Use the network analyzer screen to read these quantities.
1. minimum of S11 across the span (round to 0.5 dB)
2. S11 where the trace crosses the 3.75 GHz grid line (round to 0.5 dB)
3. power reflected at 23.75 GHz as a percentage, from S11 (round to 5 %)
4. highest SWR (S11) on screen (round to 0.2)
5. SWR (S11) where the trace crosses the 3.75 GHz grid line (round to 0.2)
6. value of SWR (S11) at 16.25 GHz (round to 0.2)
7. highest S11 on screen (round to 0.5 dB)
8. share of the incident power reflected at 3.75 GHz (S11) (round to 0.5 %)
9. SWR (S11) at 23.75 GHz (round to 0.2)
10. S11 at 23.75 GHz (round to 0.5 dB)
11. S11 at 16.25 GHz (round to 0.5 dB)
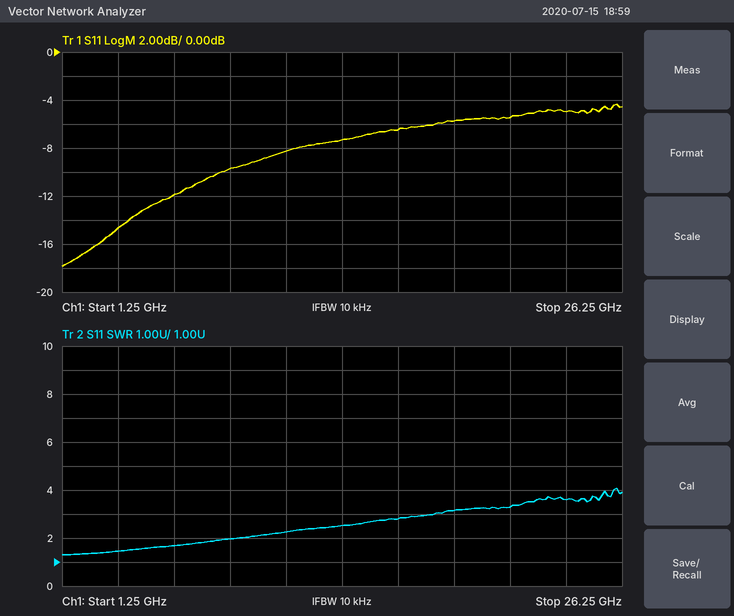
-18.0 dB
-14.5 dB
30 %
4.0
1.4
2.8
-4.5 dB
3.5 %
3.6
-5.0 dB
-6.5 dB
